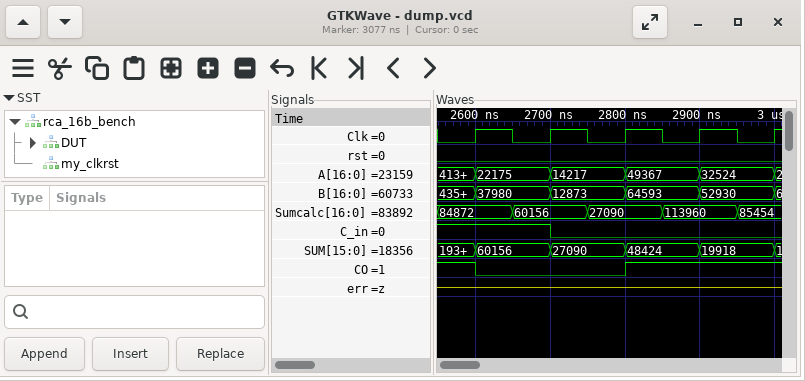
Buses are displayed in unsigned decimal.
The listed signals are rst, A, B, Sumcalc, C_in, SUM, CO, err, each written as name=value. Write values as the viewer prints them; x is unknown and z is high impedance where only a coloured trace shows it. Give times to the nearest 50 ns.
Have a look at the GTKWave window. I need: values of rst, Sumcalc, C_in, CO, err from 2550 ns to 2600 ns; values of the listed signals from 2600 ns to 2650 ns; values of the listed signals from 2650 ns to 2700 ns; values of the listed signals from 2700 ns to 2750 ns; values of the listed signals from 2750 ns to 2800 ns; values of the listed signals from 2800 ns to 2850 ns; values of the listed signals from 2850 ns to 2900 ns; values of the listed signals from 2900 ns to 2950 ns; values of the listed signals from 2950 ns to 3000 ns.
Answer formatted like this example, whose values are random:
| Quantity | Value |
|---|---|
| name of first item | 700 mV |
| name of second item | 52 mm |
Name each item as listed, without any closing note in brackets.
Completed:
| Quantity | Value |
|---|---|
| values of rst, Sumcalc, C_in, CO, err from 2550 ns to 2600 ns | rst=0, Sumcalc=84872, C_in=1, CO=1, err=z |
| values of the listed signals from 2600 ns to 2650 ns | rst=0, A=22175, B=37980, Sumcalc=84872, C_in=1, SUM=60156, CO=0, err=z |
| values of the listed signals from 2650 ns to 2700 ns | rst=0, A=22175, B=37980, Sumcalc=60156, C_in=1, SUM=60156, CO=0, err=z |
| values of the listed signals from 2700 ns to 2750 ns | rst=0, A=14217, B=12873, Sumcalc=60156, C_in=0, SUM=27090, CO=0, err=z |
| values of the listed signals from 2750 ns to 2800 ns | rst=0, A=14217, B=12873, Sumcalc=27090, C_in=0, SUM=27090, CO=0, err=z |
| values of the listed signals from 2800 ns to 2850 ns | rst=0, A=49367, B=64593, Sumcalc=27090, C_in=0, SUM=48424, CO=1, err=z |
| values of the listed signals from 2850 ns to 2900 ns | rst=0, A=49367, B=64593, Sumcalc=113960, C_in=0, SUM=48424, CO=1, err=z |
| values of the listed signals from 2900 ns to 2950 ns | rst=0, A=32524, B=52930, Sumcalc=113960, C_in=0, SUM=19918, CO=1, err=z |
| values of the listed signals from 2950 ns to 3000 ns | rst=0, A=32524, B=52930, Sumcalc=85454, C_in=0, SUM=19918, CO=1, err=z |
